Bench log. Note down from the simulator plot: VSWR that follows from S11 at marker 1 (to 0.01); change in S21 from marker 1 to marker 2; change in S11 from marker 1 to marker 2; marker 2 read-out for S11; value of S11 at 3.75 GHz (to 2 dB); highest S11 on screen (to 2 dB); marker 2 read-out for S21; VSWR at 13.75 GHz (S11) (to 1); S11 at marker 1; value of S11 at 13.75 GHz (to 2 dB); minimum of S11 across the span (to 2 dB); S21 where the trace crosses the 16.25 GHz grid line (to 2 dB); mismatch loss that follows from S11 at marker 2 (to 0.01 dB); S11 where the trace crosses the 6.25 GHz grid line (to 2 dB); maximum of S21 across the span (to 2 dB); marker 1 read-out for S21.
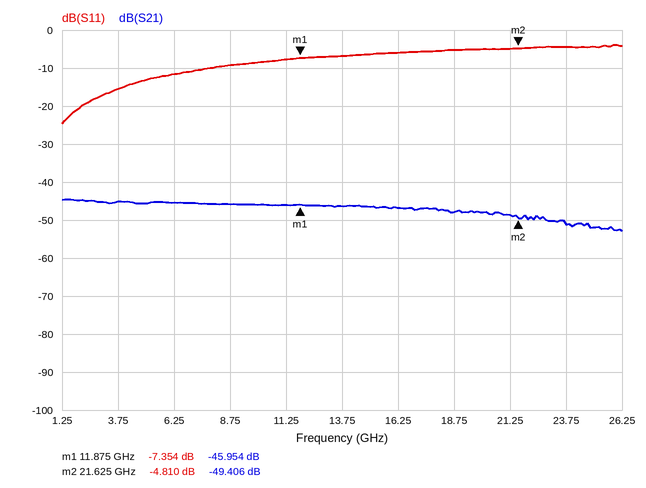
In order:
2.50
-3.452 dB
2.544 dB
-4.810 dB
-16 dB
-4 dB
-49.406 dB
3
-7.354 dB
-6 dB
-24 dB
-46 dB
1.74 dB
-12 dB
-44 dB
-45.954 dB
